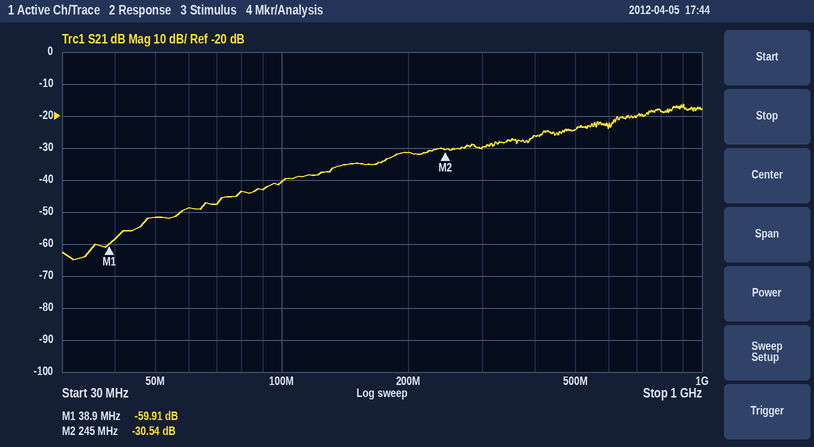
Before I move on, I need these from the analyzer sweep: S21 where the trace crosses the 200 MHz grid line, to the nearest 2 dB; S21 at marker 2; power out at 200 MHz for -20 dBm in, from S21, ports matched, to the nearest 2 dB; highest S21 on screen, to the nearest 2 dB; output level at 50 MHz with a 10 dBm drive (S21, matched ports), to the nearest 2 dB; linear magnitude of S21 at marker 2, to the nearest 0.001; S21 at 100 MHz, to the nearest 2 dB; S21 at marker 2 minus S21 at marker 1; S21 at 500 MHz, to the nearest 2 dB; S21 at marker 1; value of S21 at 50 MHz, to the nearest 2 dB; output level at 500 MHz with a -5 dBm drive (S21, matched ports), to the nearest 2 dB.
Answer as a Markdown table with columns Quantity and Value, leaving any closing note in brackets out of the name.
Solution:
| Quantity | Value |
|---|---|
| S21 where the trace crosses the 200 MHz grid line, to the nearest 2 dB | -32 dB |
| S21 at marker 2 | -30.54 dB |
| power out at 200 MHz for -20 dBm in, from S21, ports matched, to the nearest 2 dB | -52 dBm |
| highest S21 on screen, to the nearest 2 dB | -16 dB |
| output level at 50 MHz with a 10 dBm drive (S21, matched ports), to the nearest 2 dB | -42 dBm |
| linear magnitude of S21 at marker 2, to the nearest 0.001 | 0.030 |
| S21 at 100 MHz, to the nearest 2 dB | -40 dB |
| S21 at marker 2 minus S21 at marker 1 | 29.37 dB |
| S21 at 500 MHz, to the nearest 2 dB | -24 dB |
| S21 at marker 1 | -59.91 dB |
| value of S21 at 50 MHz, to the nearest 2 dB | -52 dB |
| output level at 500 MHz with a -5 dBm drive (S21, matched ports), to the nearest 2 dB | -30 dBm |
